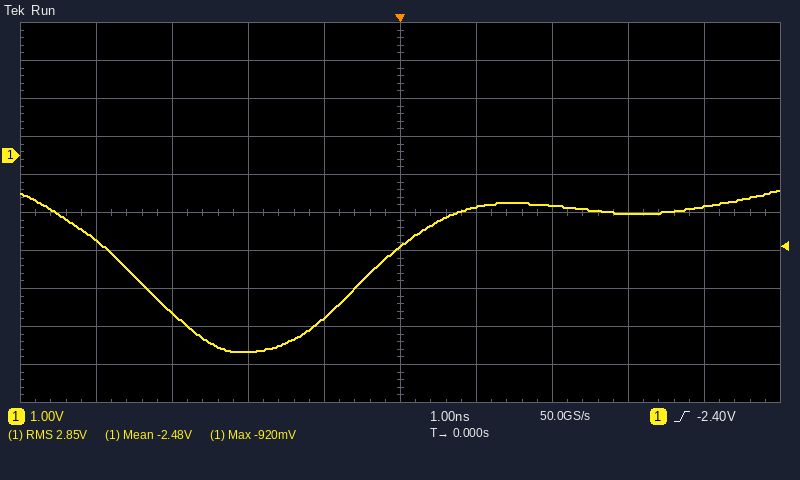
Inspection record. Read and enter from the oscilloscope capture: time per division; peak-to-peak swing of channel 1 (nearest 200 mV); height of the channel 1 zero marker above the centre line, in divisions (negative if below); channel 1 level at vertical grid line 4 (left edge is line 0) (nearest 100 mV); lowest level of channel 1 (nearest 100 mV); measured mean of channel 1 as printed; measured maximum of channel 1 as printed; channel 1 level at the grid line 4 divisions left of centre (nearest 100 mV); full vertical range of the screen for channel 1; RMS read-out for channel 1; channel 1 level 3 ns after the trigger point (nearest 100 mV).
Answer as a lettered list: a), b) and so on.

a) 1 ns
b) 4.2 V
c) +1.5 div
d) -4.3 V
e) -5.2 V
f) -2.48 V
g) -920 mV
h) -2.2 V
i) 10 V
j) 2.85 V
k) -1.5 V
